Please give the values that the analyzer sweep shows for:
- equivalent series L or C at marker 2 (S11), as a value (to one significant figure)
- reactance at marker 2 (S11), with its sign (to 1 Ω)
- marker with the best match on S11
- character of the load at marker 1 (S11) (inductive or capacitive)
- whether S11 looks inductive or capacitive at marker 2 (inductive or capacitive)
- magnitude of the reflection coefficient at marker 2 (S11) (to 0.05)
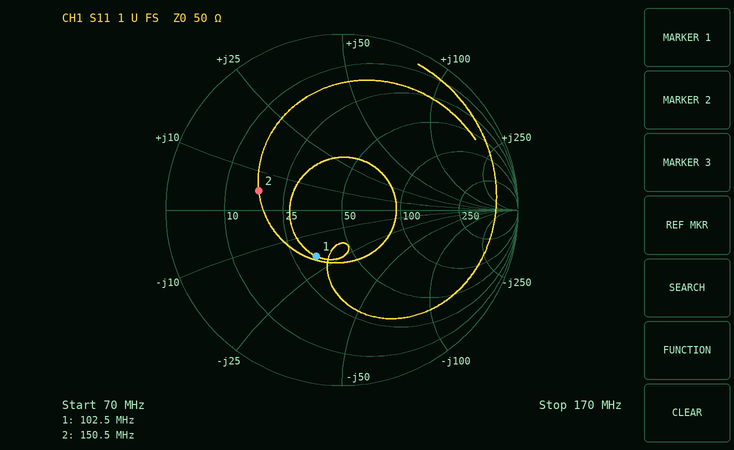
5 nH
+5 Ω
marker 1
capacitive
inductive
0.50
